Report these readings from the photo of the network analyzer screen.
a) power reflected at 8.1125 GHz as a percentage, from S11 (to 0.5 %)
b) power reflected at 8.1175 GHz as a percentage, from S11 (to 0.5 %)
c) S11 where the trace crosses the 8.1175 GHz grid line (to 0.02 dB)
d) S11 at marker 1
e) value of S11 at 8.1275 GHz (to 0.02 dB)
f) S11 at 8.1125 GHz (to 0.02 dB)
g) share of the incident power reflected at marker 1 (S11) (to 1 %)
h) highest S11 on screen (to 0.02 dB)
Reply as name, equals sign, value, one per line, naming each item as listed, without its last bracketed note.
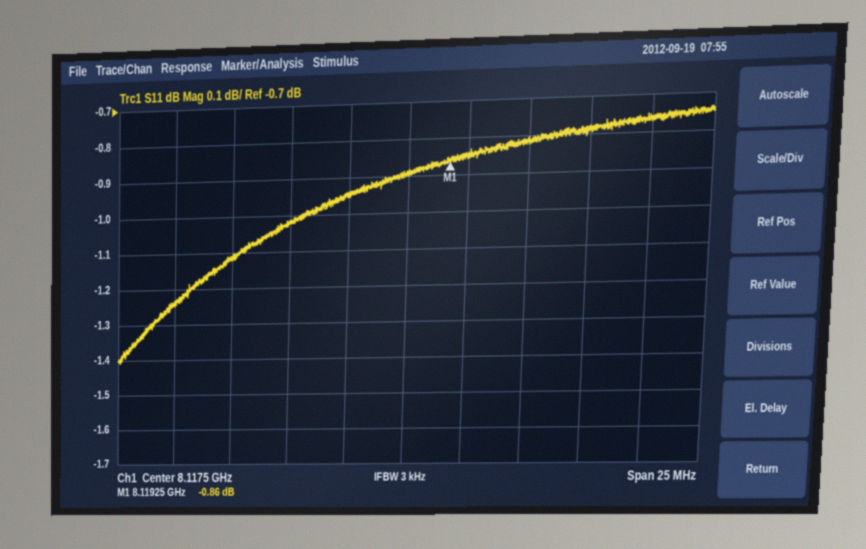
power reflected at 8.1125 GHz as a percentage, from S11 = 79.0 %
power reflected at 8.1175 GHz as a percentage, from S11 = 81.5 %
S11 where the trace crosses the 8.1175 GHz grid line = -0.90 dB
S11 at marker 1 = -0.86 dB
value of S11 at 8.1275 GHz = -0.76 dB
S11 at 8.1125 GHz = -1.02 dB
share of the incident power reflected at marker 1 (S11) = 82 %
highest S11 on screen = -0.74 dB
